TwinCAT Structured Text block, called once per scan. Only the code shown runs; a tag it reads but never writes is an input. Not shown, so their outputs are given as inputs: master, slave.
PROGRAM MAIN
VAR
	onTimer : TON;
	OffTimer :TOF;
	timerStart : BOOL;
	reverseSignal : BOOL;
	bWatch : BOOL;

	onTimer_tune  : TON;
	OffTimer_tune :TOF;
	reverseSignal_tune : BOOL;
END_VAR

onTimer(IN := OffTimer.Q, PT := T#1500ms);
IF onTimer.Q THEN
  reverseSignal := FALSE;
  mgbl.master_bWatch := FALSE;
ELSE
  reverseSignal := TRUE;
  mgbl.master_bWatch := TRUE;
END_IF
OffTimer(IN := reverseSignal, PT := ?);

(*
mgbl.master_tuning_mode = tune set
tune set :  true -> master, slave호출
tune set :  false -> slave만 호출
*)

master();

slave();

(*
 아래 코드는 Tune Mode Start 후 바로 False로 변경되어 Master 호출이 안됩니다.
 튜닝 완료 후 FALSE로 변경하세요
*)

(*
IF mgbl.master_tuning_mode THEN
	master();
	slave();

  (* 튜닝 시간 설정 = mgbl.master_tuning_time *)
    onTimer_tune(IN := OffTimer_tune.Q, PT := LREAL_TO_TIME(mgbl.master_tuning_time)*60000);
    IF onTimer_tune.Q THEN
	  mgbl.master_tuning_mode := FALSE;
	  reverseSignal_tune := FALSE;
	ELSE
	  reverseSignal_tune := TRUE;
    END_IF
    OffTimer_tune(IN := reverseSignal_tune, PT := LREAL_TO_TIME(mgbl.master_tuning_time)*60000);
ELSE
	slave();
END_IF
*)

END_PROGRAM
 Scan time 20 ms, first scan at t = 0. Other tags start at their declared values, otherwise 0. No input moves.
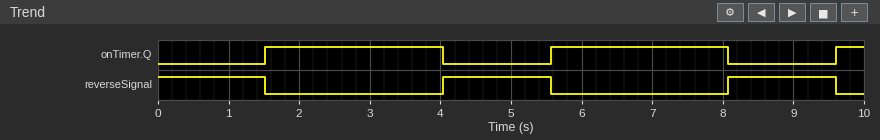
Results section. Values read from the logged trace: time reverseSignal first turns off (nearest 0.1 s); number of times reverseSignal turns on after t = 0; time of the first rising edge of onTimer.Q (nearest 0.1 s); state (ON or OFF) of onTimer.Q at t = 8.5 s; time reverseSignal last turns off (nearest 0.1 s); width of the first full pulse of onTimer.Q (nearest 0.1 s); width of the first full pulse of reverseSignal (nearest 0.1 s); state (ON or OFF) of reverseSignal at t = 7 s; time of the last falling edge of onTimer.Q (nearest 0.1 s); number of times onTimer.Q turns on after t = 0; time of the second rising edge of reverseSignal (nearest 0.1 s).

1.5 s
2
1.5 s
OFF
9.6 s
2.5 s
1.5 s
OFF
8.1 s
3
8.1 s
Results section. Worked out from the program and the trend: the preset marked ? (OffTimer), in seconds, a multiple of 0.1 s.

2.5 s
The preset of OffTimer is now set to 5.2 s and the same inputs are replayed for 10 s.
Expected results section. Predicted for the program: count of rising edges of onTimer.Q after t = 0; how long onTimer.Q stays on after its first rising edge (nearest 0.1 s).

2
5.2 s
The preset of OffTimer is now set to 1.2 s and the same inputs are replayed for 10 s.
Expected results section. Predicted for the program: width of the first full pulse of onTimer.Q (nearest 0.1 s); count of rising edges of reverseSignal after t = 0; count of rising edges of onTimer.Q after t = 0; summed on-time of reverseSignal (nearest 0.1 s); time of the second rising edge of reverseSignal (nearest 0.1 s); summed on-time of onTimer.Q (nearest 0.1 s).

1.2 s
3
4
6.1 s
5.5 s
3.9 s
